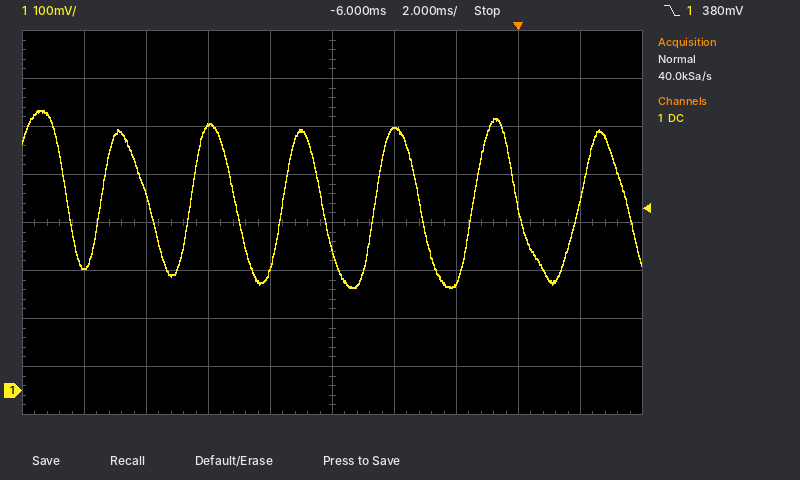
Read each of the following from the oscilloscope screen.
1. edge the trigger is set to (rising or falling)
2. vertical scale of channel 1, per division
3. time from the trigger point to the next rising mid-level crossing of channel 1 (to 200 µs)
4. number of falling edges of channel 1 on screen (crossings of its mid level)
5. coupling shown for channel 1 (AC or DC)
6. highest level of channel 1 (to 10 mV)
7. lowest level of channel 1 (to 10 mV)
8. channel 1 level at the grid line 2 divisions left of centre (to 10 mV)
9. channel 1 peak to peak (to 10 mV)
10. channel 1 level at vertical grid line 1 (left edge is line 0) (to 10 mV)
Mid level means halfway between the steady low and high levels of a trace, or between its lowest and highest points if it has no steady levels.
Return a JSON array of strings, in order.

["falling", "100 mV", "2.0 ms", "7", "DC", "580 mV", "210 mV", "550 mV", "370 mV", "260 mV"]
